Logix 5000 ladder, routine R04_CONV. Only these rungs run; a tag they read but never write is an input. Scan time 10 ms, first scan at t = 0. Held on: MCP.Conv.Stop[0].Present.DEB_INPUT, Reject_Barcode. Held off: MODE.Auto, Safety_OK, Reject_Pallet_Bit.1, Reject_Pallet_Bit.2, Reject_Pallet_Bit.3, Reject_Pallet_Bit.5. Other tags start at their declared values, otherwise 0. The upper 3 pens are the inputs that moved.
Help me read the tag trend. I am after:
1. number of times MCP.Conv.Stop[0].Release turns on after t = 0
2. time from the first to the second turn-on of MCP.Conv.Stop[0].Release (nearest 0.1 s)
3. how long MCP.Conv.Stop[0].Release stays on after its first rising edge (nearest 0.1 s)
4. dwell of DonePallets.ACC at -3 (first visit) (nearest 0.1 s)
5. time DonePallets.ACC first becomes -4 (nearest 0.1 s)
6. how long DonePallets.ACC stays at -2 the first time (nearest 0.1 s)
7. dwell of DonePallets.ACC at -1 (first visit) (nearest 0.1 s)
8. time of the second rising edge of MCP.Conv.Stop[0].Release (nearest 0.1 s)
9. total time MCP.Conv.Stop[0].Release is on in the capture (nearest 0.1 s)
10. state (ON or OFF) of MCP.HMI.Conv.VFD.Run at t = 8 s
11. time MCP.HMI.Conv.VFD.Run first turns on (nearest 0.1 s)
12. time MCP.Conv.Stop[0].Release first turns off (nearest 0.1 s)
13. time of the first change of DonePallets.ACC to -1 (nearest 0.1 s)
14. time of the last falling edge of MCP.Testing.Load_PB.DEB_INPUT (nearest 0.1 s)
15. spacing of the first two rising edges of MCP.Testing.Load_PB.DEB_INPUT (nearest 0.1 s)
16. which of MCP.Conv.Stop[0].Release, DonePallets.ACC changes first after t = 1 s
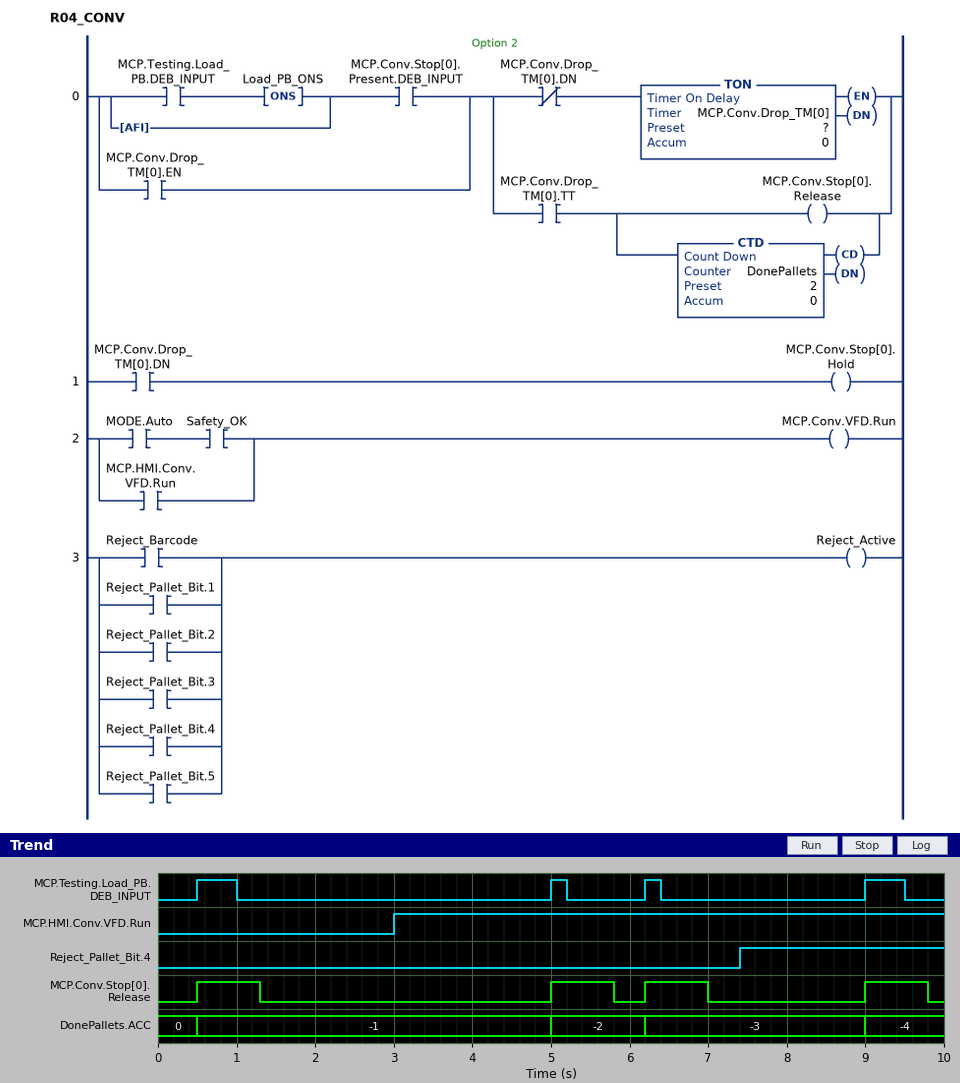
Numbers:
4
4.5 s
0.8 s
2.8 s
9.0 s
1.2 s
4.5 s
5.0 s
3.2 s
ON
3.0 s
1.3 s
0.5 s
9.5 s
4.5 s
MCP.Conv.Stop[0].Release
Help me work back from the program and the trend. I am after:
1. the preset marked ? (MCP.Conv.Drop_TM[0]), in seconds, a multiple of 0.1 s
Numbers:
0.8 s
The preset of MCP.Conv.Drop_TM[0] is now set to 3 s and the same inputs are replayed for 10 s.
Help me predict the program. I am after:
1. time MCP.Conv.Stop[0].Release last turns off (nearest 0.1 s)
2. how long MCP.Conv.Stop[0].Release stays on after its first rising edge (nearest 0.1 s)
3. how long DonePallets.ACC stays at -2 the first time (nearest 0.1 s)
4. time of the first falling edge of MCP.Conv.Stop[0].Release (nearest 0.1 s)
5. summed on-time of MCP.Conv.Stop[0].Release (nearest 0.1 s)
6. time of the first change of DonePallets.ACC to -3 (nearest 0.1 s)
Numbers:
8.0 s
3.0 s
4.0 s
3.5 s
7.0 s
9.0 s
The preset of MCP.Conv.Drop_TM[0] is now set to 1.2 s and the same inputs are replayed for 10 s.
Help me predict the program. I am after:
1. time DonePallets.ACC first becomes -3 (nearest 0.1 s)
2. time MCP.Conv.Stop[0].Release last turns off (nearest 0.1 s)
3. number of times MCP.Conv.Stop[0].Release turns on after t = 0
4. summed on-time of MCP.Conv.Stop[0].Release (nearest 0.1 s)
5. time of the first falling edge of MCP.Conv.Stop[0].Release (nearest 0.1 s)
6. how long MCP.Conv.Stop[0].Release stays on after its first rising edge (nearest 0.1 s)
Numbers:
9.0 s
6.2 s
3
3.4 s
1.7 s
1.2 s
